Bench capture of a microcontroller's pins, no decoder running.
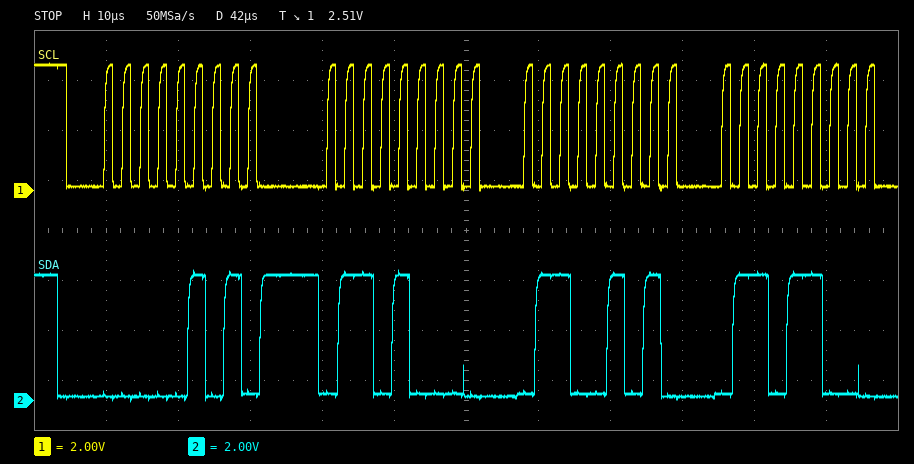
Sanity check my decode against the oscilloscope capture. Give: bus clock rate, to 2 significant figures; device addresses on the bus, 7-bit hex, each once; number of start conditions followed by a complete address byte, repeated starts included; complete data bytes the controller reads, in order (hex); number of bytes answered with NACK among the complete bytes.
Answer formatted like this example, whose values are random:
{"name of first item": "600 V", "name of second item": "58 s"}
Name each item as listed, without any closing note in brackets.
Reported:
{"bus clock rate, to 2 significant figures": "400 kHz", "device addresses on the bus, 7-bit hex, each once": "0x02", "number of start conditions followed by a complete address byte, repeated starts included": "1", "complete data bytes the controller reads, in order": "68 65 6C", "number of bytes answered with NACK among the complete bytes": "0"}
